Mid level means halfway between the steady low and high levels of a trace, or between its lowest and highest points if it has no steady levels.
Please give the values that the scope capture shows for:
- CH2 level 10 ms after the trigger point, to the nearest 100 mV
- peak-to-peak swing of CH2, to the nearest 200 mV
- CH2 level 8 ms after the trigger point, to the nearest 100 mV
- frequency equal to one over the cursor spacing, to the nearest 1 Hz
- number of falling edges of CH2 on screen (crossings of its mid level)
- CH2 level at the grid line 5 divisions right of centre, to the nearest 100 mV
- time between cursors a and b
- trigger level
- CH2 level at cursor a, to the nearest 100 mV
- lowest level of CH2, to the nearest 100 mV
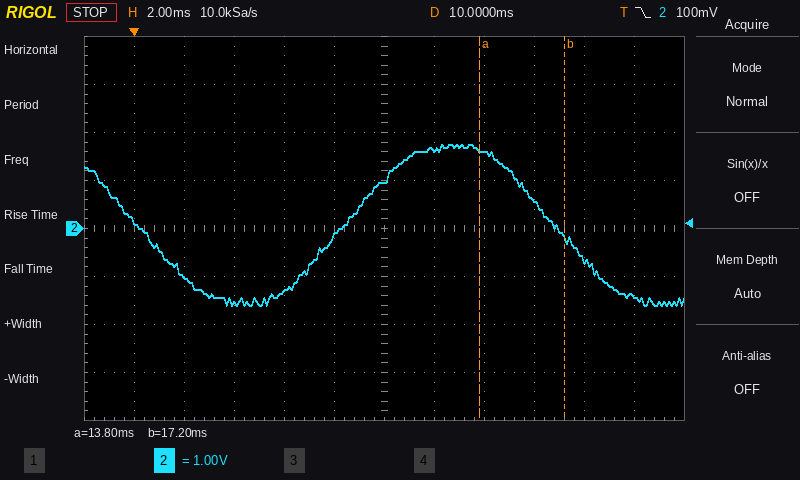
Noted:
1.0 V
3.4 V
-200 mV
294 Hz
2
-1.4 V
3.4 ms
100 mV
1.6 V
-1.6 V
